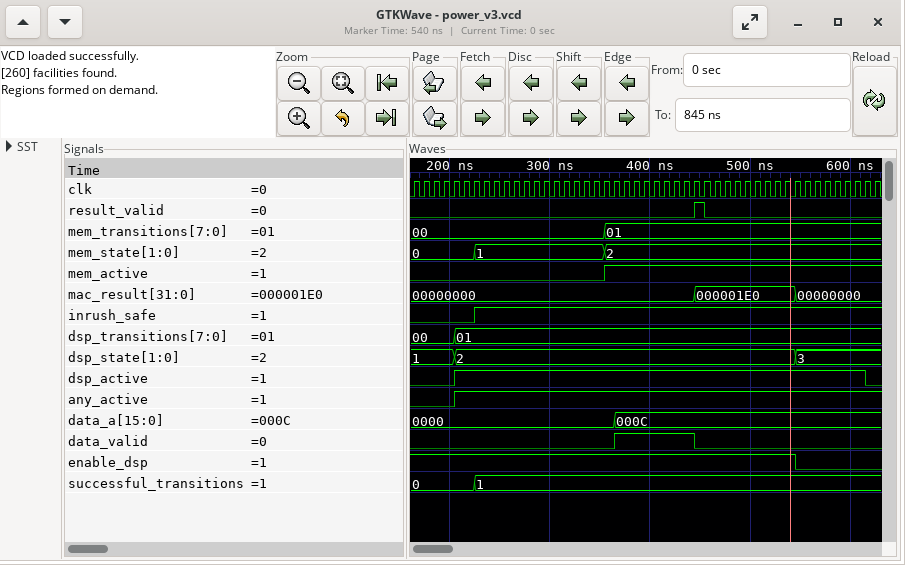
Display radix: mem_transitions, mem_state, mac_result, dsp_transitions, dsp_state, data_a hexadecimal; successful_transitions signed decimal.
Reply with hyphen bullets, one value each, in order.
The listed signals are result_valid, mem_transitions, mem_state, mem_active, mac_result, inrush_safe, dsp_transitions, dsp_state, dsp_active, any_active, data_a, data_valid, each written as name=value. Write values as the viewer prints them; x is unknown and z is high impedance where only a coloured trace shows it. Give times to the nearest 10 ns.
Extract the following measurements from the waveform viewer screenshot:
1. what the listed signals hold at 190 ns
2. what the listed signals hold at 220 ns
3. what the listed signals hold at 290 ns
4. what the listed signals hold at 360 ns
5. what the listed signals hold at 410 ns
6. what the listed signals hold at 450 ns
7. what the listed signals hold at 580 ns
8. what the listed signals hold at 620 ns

- result_valid=0, mem_transitions=00, mem_state=0, mem_active=0, mac_result=00000000, inrush_safe=0, dsp_transitions=00, dsp_state=1, dsp_active=0, any_active=0, data_a=0000, data_valid=0
- result_valid=0, mem_transitions=00, mem_state=0, mem_active=0, mac_result=00000000, inrush_safe=0, dsp_transitions=01, dsp_state=2, dsp_active=1, any_active=1, data_a=0000, data_valid=0
- result_valid=0, mem_transitions=00, mem_state=1, mem_active=0, mac_result=00000000, inrush_safe=1, dsp_transitions=01, dsp_state=2, dsp_active=1, any_active=1, data_a=0000, data_valid=0
- result_valid=0, mem_transitions=01, mem_state=2, mem_active=1, mac_result=00000000, inrush_safe=1, dsp_transitions=01, dsp_state=2, dsp_active=1, any_active=1, data_a=0000, data_valid=0
- result_valid=0, mem_transitions=01, mem_state=2, mem_active=1, mac_result=00000000, inrush_safe=1, dsp_transitions=01, dsp_state=2, dsp_active=1, any_active=1, data_a=000C, data_valid=1
- result_valid=1, mem_transitions=01, mem_state=2, mem_active=1, mac_result=000001E0, inrush_safe=1, dsp_transitions=01, dsp_state=2, dsp_active=1, any_active=1, data_a=000C, data_valid=0
- result_valid=0, mem_transitions=01, mem_state=2, mem_active=1, mac_result=00000000, inrush_safe=1, dsp_transitions=01, dsp_state=3, dsp_active=1, any_active=1, data_a=000C, data_valid=0
- result_valid=0, mem_transitions=01, mem_state=2, mem_active=1, mac_result=00000000, inrush_safe=1, dsp_transitions=01, dsp_state=3, dsp_active=0, any_active=1, data_a=000C, data_valid=0
